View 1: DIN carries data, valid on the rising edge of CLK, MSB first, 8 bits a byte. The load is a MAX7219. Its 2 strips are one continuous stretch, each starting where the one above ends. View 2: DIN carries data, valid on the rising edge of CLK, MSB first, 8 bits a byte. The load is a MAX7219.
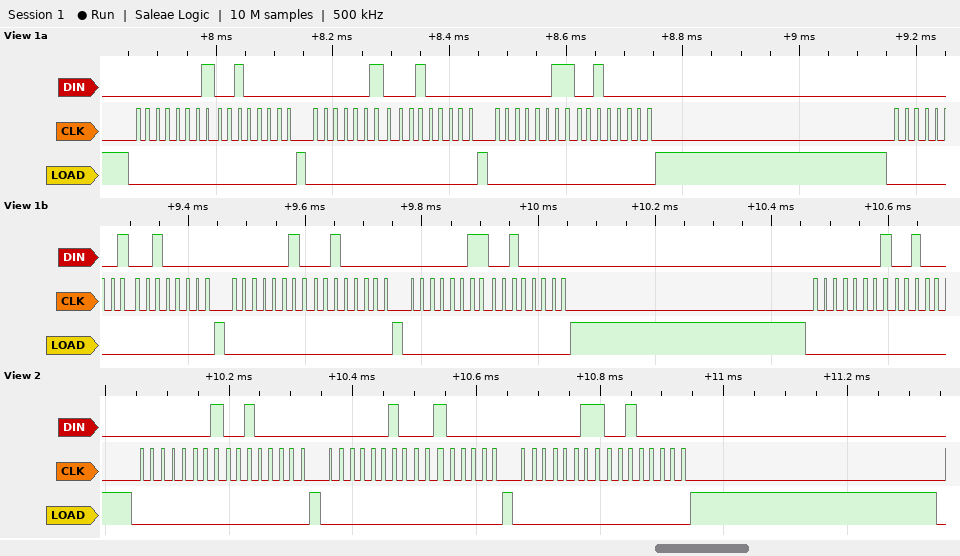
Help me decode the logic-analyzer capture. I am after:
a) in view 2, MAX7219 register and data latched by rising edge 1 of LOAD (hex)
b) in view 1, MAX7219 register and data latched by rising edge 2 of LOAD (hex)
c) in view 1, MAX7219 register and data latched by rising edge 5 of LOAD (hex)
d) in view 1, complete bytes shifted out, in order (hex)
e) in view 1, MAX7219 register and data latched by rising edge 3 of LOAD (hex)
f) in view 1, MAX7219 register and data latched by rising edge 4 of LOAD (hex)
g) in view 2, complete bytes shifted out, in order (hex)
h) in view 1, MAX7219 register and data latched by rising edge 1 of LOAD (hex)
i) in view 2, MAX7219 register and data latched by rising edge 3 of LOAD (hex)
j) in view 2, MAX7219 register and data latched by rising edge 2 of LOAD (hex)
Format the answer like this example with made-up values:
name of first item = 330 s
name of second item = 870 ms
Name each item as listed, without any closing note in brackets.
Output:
in view 2, MAX7219 register and data latched by rising edge 1 of LOAD = register 0x1, data 0x20
in view 1, MAX7219 register and data latched by rising edge 2 of LOAD = register 0x2, data 0x20
in view 1, MAX7219 register and data latched by rising edge 5 of LOAD = register 0x2, data 0x20
in view 1, complete bytes shifted out, in order = 0x01 0x20 0x02 0x20 0x03 0x20 0x01 0x20 0x02 0x20 0x03 0x20 0x01
in view 1, MAX7219 register and data latched by rising edge 3 of LOAD = register 0x3, data 0x20
in view 1, MAX7219 register and data latched by rising edge 4 of LOAD = register 0x1, data 0x20
in view 2, complete bytes shifted out, in order = 01 20 02 20 03 20
in view 1, MAX7219 register and data latched by rising edge 1 of LOAD = register 0x1, data 0x20
in view 2, MAX7219 register and data latched by rising edge 3 of LOAD = register 0x3, data 0x20
in view 2, MAX7219 register and data latched by rising edge 2 of LOAD = register 0x2, data 0x20
